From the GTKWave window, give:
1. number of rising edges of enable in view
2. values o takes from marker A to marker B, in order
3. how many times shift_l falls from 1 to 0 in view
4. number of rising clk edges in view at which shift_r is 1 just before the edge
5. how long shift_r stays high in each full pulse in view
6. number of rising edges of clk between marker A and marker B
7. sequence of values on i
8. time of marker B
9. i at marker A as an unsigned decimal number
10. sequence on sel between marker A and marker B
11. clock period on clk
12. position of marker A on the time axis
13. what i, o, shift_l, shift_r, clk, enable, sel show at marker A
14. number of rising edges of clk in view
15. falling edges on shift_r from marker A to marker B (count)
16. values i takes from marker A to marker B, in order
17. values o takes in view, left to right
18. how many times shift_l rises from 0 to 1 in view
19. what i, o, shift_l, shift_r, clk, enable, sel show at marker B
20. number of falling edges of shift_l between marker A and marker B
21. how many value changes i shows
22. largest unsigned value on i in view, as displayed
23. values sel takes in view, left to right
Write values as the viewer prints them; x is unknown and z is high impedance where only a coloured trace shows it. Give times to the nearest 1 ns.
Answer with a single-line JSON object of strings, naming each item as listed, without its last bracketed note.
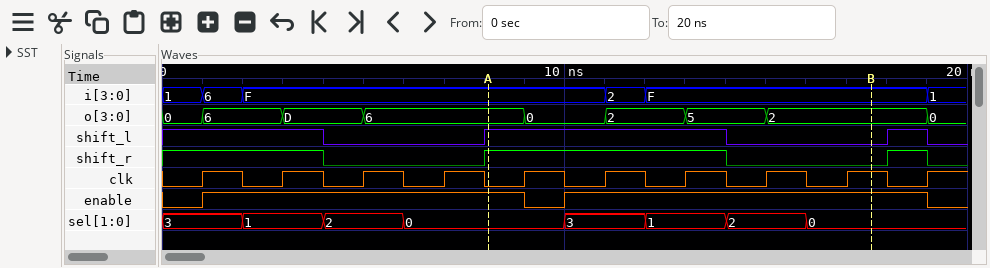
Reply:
{"number of rising edges of enable in view": "2", "values o takes from marker A to marker B, in order": "6, 0, 2, 5, 2", "how many times shift_l falls from 1 to 0 in view": "3", "number of rising clk edges in view at which shift_r is 1 just before the edge": "6", "how long shift_r stays high in each full pulse in view": "6 ns, 1 ns", "number of rising edges of clk between marker A and marker B": "5", "sequence of values on i": "1, 6, F, 2, F, 1", "time of marker B": "18 ns", "i at marker A as an unsigned decimal number": "15", "sequence on sel between marker A and marker B": "0, 3, 1, 2, 0", "clock period on clk": "2 ns", "position of marker A on the time axis": "8 ns", "what i, o, shift_l, shift_r, clk, enable, sel show at marker A": "i=F, o=6, shift_l=1, shift_r=1, clk=0, enable=1, sel=0", "number of rising edges of clk in view": "10", "falling edges on shift_r from marker A to marker B": "1", "values i takes from marker A to marker B, in order": "F, 2, F", "values o takes in view, left to right": "0, 6, D, 6, 0, 2, 5, 2, 0", "how many times shift_l rises from 0 to 1 in view": "2", "what i, o, shift_l, shift_r, clk, enable, sel show at marker B": "i=F, o=2, shift_l=0, shift_r=0, clk=1, enable=1, sel=0", "number of falling edges of shift_l between marker A and marker B": "1", "how many value changes i shows": "5", "largest unsigned value on i in view, as displayed": "F", "values sel takes in view, left to right": "3, 1, 2, 0, 3, 1, 2, 0"}
